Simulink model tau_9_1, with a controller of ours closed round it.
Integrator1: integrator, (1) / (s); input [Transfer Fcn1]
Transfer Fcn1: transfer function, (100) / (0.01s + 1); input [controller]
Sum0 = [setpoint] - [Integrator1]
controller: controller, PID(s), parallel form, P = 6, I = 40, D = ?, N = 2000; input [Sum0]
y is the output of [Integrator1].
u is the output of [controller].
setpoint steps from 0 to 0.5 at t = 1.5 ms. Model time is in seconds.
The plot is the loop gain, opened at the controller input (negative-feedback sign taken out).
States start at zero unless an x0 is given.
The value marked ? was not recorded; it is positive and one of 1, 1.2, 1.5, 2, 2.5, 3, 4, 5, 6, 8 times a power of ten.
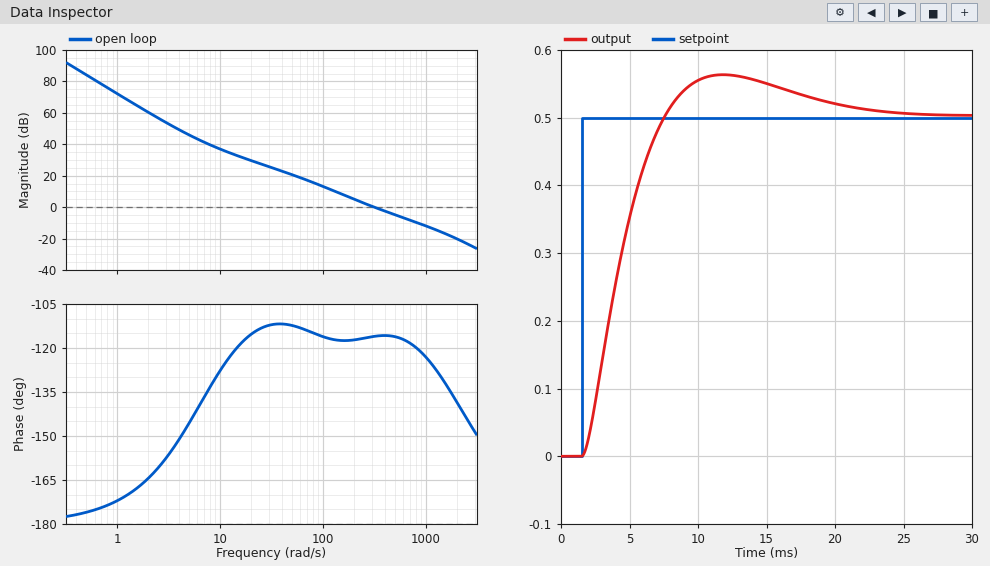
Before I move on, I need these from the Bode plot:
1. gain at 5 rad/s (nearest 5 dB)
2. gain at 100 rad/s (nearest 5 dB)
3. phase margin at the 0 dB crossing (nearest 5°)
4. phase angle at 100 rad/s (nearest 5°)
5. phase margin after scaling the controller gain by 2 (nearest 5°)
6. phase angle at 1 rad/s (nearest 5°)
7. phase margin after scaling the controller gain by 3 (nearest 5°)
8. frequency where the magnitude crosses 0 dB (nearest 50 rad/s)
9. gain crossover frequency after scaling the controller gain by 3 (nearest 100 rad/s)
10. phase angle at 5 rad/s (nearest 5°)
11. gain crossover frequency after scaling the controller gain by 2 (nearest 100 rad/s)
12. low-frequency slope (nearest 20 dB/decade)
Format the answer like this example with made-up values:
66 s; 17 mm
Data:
45 dB; 15 dB; 65°; -115°; 65°; -170°; 60°; 300 rad/s; 800 rad/s; -145°; 600 rad/s; -40 dB/decade
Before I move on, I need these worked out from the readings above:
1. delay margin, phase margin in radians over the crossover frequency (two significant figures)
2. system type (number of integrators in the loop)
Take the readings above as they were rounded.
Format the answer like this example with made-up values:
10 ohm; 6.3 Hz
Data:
0.0038 s; 2
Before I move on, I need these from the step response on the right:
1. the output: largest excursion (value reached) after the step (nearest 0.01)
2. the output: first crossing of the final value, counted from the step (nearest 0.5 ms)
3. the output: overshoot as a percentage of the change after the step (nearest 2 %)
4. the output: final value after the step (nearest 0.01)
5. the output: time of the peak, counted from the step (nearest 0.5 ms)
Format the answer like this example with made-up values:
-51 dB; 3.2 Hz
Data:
0.56; 6.0 ms; 12 %; 0.50; 10.5 ms
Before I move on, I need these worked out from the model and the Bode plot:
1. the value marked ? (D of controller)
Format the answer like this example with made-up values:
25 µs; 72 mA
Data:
0.025
